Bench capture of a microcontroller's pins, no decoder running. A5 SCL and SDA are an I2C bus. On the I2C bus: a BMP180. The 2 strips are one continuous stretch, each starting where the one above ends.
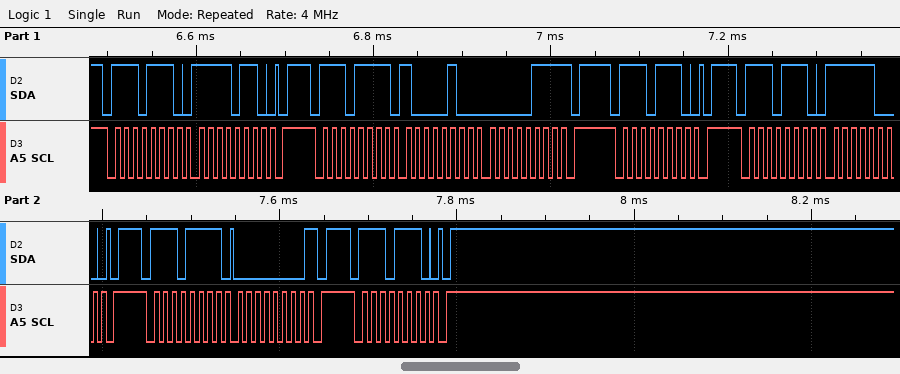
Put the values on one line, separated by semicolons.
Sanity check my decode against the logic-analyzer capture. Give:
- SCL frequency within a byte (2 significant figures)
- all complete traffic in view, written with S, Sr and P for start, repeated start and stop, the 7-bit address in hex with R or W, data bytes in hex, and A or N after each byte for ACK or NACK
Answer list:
100 kHz; S 77W A F6 A P S 77R A 84 A 07 N P S 77W A P S 77W A F8 A P S 77R A 00 N P S 77W A P
